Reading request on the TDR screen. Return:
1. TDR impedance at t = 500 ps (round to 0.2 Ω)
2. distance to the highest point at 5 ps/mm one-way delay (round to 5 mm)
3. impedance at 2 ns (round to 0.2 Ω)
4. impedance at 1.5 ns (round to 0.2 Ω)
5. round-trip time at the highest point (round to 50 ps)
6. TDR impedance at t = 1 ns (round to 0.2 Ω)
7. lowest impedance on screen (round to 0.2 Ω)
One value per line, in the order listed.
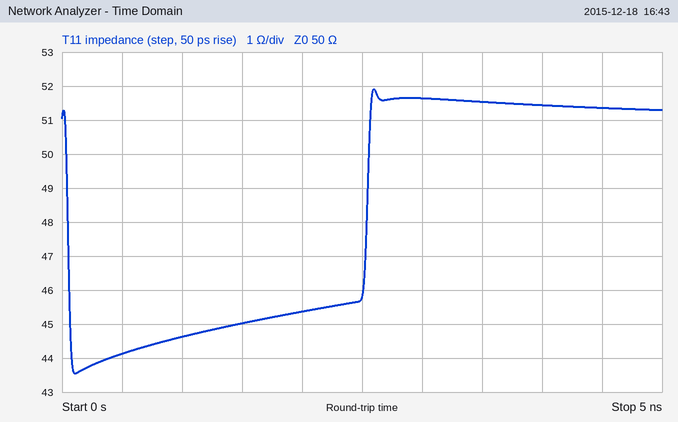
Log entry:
44.2 Ω
260 mm
45.4 Ω
45.0 Ω
2.60 ns
44.6 Ω
43.6 Ω
